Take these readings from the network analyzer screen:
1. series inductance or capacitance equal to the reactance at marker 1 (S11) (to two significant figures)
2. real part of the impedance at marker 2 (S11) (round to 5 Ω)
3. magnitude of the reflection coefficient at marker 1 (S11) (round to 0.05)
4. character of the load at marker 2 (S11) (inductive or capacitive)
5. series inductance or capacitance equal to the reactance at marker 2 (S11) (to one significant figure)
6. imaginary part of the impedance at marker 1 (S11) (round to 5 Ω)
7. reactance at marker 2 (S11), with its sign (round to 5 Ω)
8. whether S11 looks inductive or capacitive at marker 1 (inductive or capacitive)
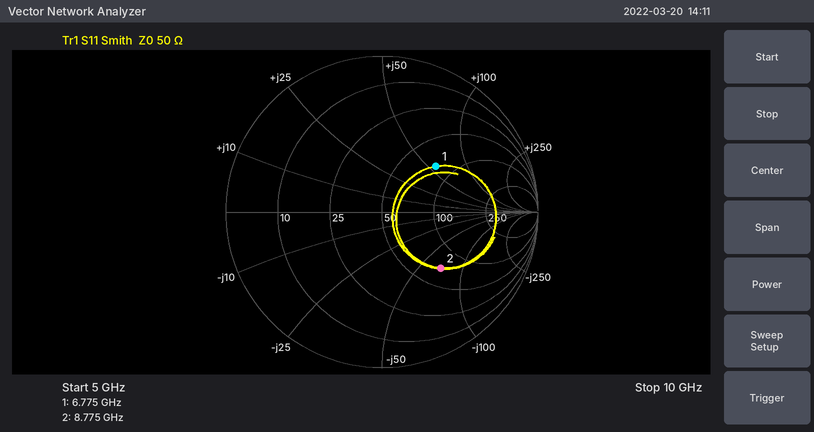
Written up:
1.3 nH
70 Ω
0.45
capacitive
300 fF
+55 Ω
-70 Ω
inductive
